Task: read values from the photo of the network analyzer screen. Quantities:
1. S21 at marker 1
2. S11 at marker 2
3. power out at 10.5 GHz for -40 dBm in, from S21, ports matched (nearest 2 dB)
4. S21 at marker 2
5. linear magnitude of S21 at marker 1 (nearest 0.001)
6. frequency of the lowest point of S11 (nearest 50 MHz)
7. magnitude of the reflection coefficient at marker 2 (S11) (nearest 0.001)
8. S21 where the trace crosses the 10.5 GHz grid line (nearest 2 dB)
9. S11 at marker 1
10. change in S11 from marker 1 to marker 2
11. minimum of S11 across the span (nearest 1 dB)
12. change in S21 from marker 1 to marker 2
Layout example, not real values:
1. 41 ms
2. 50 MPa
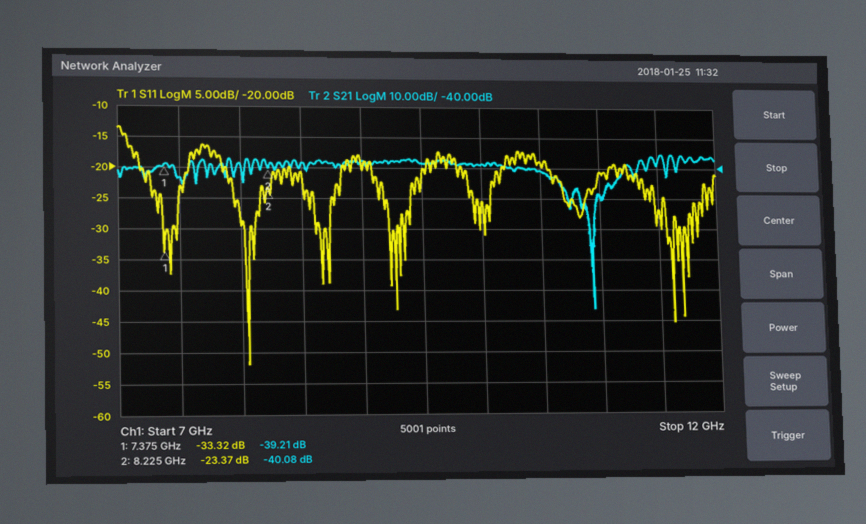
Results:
1. -39.21 dB
2. -23.37 dB
3. -80 dBm
4. -40.08 dB
5. 0.011
6. 8.05 GHz
7. 0.068
8. -40 dB
9. -33.32 dB
10. 9.95 dB
11. -52 dB
12. -0.87 dB
